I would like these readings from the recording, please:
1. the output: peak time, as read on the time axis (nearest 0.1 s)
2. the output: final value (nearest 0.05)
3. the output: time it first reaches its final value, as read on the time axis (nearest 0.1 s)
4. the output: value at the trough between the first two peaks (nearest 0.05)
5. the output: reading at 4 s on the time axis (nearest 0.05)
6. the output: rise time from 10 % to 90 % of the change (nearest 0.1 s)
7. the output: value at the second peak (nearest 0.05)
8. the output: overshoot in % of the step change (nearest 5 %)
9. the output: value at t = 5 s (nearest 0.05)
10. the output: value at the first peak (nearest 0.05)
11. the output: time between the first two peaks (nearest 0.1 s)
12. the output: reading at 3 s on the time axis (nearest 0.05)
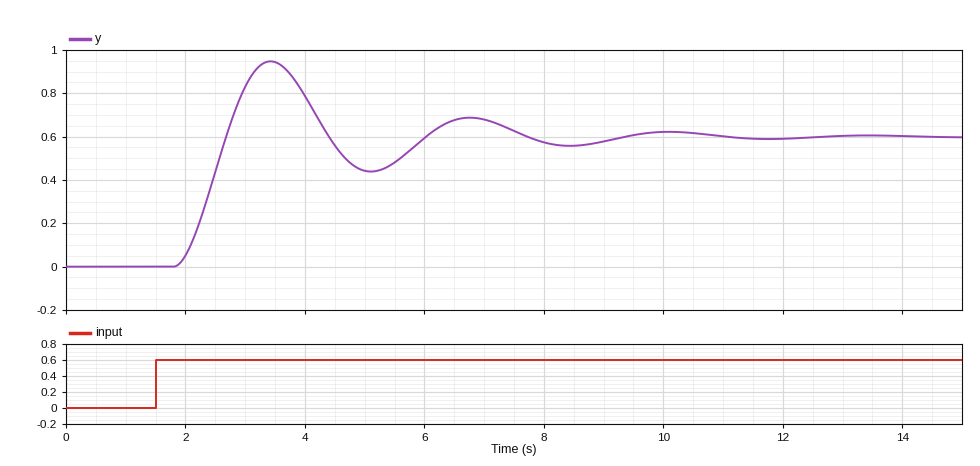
3.4 s
0.60
2.7 s
0.45
0.80
0.6 s
0.70
60 %
0.45
0.95
3.3 s
0.85
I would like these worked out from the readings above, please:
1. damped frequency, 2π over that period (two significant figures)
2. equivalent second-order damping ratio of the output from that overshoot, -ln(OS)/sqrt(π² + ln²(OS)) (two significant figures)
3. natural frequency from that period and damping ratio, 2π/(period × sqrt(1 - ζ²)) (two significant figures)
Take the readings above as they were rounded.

1.9 rad/s
0.16
1.9 rad/s
